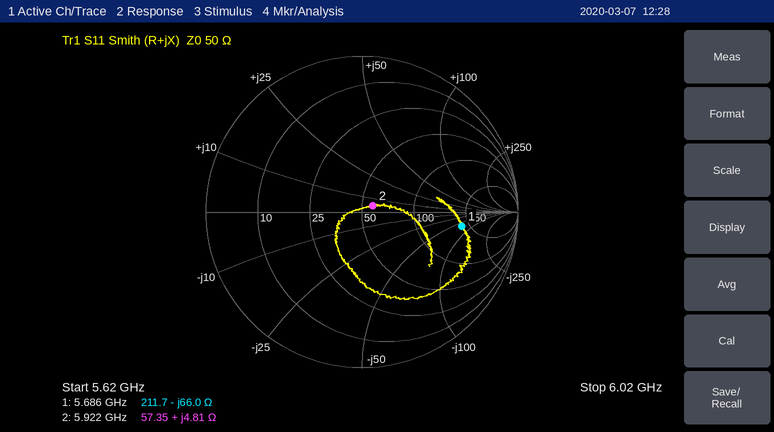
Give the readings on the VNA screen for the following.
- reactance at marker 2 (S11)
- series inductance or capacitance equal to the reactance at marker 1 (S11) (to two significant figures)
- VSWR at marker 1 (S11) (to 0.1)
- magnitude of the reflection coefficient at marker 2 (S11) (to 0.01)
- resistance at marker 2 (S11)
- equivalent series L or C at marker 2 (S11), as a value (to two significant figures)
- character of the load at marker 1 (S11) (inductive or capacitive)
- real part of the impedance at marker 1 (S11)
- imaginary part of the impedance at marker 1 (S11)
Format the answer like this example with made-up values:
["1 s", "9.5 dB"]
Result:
["+4.81 Ω", "420 fF", "4.7", "0.08", "57.35 Ω", "130 pH", "capacitive", "211.7 Ω", "-66.0 Ω"]
